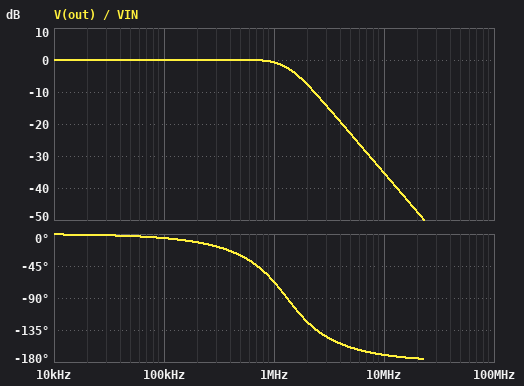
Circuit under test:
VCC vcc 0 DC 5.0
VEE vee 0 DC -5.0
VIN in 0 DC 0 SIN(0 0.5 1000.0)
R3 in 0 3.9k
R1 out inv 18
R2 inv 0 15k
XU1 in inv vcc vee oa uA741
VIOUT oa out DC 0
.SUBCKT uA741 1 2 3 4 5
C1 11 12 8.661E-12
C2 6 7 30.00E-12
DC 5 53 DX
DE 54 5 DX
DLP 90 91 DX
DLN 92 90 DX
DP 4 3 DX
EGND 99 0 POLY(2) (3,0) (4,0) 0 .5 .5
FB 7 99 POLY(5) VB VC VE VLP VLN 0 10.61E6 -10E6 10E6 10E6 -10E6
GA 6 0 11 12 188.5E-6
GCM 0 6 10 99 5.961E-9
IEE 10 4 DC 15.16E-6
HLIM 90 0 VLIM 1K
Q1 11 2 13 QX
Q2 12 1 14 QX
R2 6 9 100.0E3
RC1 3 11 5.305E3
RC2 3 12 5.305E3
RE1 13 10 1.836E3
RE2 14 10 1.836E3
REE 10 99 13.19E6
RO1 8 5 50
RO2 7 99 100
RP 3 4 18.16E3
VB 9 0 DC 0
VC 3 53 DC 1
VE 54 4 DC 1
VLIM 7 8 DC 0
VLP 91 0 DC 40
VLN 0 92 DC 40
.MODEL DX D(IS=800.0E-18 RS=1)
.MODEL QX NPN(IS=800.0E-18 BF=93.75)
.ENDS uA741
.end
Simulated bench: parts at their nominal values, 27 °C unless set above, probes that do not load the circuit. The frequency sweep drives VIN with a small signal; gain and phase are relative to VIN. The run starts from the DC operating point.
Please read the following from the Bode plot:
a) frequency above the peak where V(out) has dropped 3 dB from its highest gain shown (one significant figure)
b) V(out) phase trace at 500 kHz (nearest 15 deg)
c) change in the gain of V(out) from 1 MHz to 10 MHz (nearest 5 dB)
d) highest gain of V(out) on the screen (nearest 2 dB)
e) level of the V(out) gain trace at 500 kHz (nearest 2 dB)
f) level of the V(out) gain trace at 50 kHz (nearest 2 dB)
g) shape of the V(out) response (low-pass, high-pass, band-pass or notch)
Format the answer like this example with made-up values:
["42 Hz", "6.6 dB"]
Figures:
["1 MHz", "-30 deg", "-35 dB", "0 dB", "0 dB", "0 dB", "low-pass"]
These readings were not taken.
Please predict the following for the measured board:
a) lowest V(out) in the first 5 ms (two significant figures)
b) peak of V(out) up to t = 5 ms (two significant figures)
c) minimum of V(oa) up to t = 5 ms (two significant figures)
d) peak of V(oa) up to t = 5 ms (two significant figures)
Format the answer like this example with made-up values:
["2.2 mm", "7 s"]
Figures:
["-500 mV", "500 mV", "-500 mV", "500 mV"]
